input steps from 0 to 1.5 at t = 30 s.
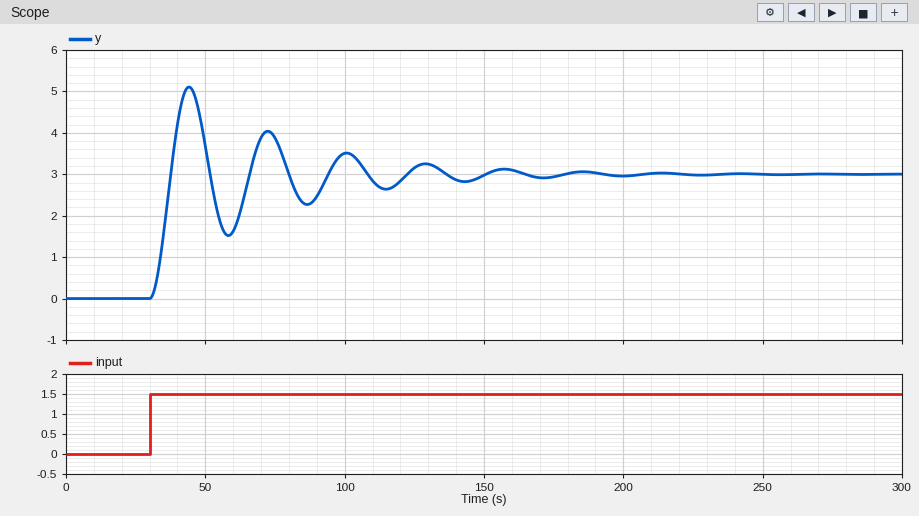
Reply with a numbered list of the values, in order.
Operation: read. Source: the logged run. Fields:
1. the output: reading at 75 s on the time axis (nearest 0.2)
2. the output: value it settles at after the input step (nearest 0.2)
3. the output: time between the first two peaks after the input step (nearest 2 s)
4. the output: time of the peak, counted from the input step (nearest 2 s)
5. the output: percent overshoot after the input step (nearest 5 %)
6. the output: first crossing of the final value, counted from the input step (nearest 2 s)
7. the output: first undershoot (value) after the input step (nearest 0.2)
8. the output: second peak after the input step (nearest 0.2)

1. 3.8
2. 3.0
3. 28 s
4. 14 s
5. 70 %
6. 8 s
7. 1.6
8. 4.0
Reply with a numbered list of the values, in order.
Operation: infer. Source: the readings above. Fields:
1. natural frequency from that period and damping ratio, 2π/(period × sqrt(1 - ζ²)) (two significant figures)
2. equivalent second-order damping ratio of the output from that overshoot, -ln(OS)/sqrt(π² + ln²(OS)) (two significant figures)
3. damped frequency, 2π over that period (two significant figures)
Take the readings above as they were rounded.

1. 0.23 rad/s
2. 0.11
3. 0.22 rad/s
